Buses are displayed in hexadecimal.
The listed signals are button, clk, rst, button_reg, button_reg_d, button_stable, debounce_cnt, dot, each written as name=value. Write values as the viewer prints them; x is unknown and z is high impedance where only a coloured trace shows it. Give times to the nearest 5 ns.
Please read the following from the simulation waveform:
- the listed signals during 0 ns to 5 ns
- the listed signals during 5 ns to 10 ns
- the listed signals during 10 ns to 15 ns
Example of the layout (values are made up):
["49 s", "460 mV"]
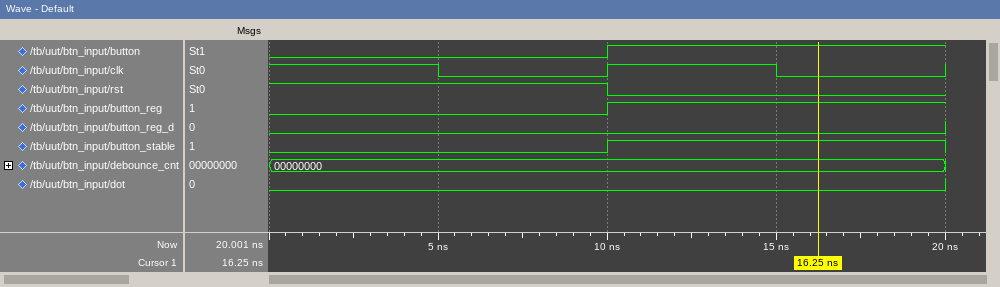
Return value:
["button=0, clk=1, rst=1, button_reg=0, button_reg_d=0, button_stable=0, debounce_cnt=00000000, dot=0", "button=0, clk=0, rst=1, button_reg=0, button_reg_d=0, button_stable=0, debounce_cnt=00000000, dot=0", "button=1, clk=1, rst=0, button_reg=1, button_reg_d=0, button_stable=1, debounce_cnt=00000000, dot=0"]
